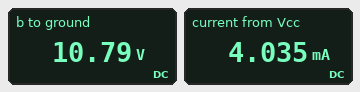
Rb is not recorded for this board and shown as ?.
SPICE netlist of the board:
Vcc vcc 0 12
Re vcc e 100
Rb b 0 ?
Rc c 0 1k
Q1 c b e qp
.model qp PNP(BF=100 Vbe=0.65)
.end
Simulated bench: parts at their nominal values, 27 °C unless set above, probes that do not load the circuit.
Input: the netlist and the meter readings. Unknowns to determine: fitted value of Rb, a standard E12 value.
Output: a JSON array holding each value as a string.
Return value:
["270 kΩ"]
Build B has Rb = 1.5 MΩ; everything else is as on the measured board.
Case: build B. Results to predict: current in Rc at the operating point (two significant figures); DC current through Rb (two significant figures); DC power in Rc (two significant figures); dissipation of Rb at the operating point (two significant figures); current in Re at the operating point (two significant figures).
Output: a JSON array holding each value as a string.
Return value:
["740 µA", "7.4 µA", "550 µW", "83 µW", "750 µA"]
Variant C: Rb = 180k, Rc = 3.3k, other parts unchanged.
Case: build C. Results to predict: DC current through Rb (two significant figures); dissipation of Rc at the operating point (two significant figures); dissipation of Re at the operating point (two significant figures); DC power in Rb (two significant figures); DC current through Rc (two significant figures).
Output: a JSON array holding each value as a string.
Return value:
["60 µA", "40 mW", "1.3 mW", "650 µW", "3.5 mA"]
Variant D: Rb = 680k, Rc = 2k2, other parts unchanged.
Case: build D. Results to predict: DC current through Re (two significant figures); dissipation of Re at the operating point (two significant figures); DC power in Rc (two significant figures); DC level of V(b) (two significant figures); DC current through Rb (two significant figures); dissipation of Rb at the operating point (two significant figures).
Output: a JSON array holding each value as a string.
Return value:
["1.6 mA", "270 µW", "5.8 mW", "11 V", "16 µA", "180 µW"]
